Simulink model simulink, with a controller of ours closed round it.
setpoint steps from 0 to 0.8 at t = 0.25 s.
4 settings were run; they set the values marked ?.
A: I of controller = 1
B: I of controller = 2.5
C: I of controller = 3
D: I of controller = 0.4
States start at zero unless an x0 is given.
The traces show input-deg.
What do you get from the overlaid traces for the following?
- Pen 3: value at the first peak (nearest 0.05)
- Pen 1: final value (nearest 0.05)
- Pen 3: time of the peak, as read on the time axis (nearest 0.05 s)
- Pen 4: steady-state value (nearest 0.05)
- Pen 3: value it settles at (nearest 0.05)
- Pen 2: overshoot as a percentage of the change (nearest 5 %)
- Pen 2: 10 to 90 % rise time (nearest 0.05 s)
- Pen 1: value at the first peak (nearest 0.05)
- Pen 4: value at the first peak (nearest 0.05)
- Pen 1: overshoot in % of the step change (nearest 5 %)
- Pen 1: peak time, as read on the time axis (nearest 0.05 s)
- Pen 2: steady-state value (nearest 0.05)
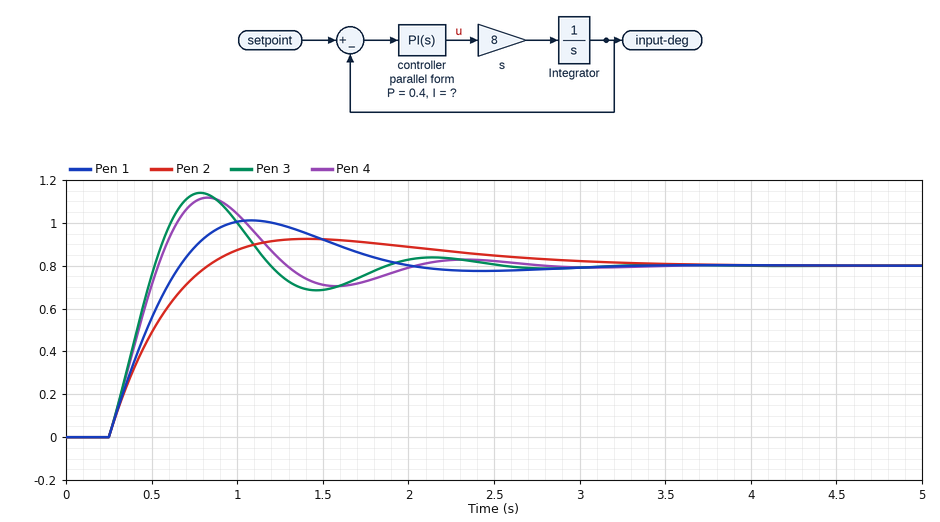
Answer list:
1.15
0.80
0.80 s
0.80
0.80
15 %
0.45 s
1.00
1.10
25 %
1.10 s
0.80
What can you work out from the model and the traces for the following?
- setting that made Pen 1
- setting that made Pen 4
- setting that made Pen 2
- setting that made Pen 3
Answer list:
A
B
D
C
